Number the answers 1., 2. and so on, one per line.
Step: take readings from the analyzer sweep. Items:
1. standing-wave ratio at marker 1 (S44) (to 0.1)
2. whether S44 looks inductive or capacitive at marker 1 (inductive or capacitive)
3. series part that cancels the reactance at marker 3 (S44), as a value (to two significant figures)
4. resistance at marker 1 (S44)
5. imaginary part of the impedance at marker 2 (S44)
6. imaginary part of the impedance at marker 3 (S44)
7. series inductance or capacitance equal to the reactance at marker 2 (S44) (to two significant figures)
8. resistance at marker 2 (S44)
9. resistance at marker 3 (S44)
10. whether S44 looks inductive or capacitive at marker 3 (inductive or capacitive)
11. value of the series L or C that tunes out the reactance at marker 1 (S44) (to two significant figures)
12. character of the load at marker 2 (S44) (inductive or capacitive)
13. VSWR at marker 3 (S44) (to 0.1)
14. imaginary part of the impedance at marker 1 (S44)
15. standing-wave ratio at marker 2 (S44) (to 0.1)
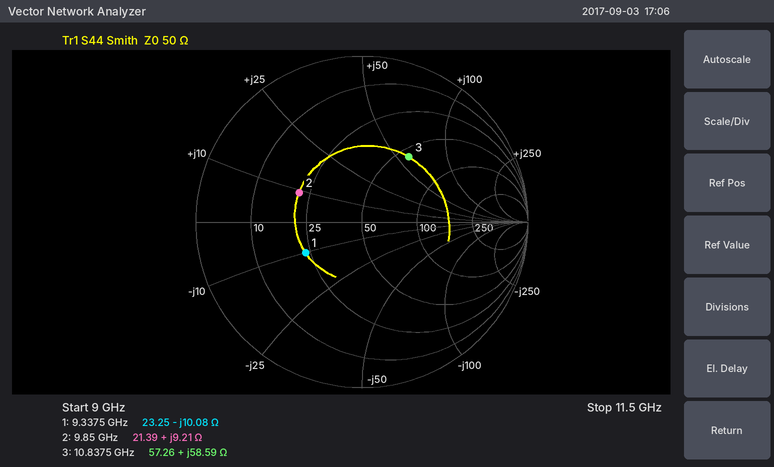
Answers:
1. 2.3
2. capacitive
3. 250 fF
4. 23.25 Ω
5. +9.21 Ω
6. +58.59 Ω
7. 150 pH
8. 21.39 Ω
9. 57.26 Ω
10. inductive
11. 170 pH
12. inductive
13. 2.9
14. -10.08 Ω
15. 2.4
